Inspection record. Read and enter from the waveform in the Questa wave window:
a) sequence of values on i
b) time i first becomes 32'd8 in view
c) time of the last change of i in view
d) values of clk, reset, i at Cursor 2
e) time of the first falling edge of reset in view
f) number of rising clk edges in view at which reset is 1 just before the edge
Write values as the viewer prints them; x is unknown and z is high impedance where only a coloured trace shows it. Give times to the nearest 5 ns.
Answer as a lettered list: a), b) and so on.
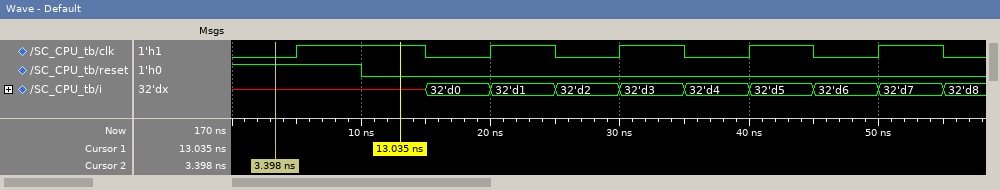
a) x, 32'd0, 32'd1, 32'd2, 32'd3, 32'd4, 32'd5, 32'd6, 32'd7, 32'd8
b) 55 ns
c) 55 ns
d) clk=0, reset=1, i=x
e) 10 ns
f) 1
